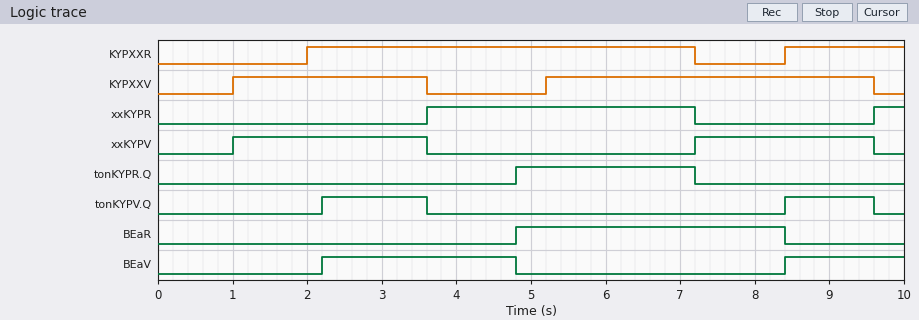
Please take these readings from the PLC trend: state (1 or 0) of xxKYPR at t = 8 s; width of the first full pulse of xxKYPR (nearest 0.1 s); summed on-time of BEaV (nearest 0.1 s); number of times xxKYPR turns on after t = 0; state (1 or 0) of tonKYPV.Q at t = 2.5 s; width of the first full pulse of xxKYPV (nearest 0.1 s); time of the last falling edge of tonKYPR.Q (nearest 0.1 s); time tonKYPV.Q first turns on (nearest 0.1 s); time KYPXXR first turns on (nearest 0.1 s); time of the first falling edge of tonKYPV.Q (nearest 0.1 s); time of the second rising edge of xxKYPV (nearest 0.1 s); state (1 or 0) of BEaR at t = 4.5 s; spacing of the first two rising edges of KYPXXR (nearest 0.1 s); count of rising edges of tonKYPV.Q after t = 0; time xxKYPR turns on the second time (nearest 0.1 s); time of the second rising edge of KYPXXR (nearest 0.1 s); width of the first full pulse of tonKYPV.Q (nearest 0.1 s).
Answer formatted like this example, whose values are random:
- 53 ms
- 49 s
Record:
- 0
- 3.6 s
- 4.2 s
- 2
- 1
- 2.6 s
- 7.2 s
- 2.2 s
- 2.0 s
- 3.6 s
- 7.2 s
- 0
- 6.4 s
- 2
- 9.6 s
- 8.4 s
- 1.4 s
